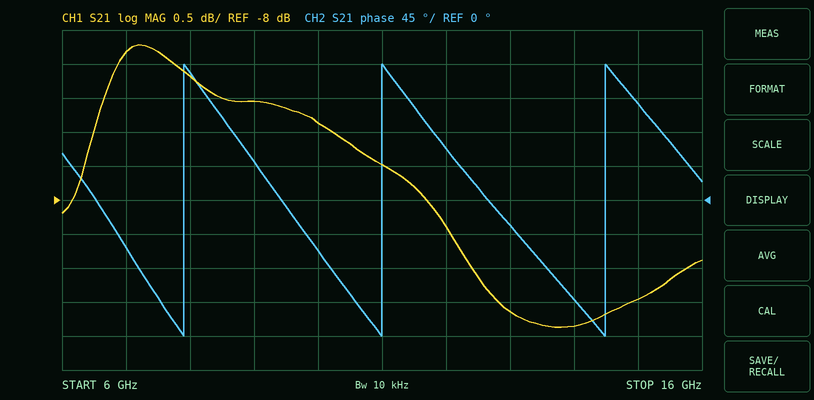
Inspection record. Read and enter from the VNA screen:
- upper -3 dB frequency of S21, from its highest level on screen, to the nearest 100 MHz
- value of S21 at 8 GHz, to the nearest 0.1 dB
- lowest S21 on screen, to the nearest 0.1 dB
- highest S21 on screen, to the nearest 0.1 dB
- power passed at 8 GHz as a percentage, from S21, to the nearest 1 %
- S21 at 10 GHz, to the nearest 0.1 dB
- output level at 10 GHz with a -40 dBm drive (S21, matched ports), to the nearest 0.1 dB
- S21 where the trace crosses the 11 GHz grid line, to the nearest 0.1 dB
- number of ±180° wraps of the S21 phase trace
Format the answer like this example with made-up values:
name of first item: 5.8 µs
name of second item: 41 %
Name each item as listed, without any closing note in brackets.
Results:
upper -3 dB frequency of S21, from its highest level on screen, to the nearest 100 MHz: 12.2 GHz
value of S21 at 8 GHz, to the nearest 0.1 dB: -6.2 dB
lowest S21 on screen, to the nearest 0.1 dB: -9.9 dB
highest S21 on screen, to the nearest 0.1 dB: -5.7 dB
power passed at 8 GHz as a percentage, from S21, to the nearest 1 %: 24 %
S21 at 10 GHz, to the nearest 0.1 dB: -6.9 dB
output level at 10 GHz with a -40 dBm drive (S21, matched ports), to the nearest 0.1 dB: -46.9 dBm
S21 where the trace crosses the 11 GHz grid line, to the nearest 0.1 dB: -7.5 dB
number of ±180° wraps of the S21 phase trace: 3
